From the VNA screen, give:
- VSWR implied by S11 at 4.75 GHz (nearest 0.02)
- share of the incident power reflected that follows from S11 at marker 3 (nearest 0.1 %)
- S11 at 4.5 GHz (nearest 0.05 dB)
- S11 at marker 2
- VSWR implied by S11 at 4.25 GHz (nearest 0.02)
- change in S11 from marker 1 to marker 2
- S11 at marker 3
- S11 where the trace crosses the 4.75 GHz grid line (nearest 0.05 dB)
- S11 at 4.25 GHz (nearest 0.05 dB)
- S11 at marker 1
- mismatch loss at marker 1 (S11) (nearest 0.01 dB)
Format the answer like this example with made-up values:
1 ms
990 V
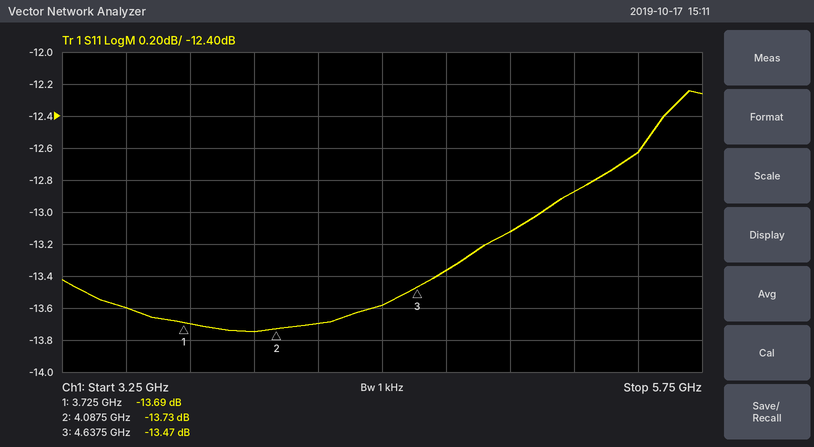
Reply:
1.54
4.5 %
-13.60 dB
-13.73 dB
1.52
-0.04 dB
-13.47 dB
-13.35 dB
-13.70 dB
-13.69 dB
0.19 dB
